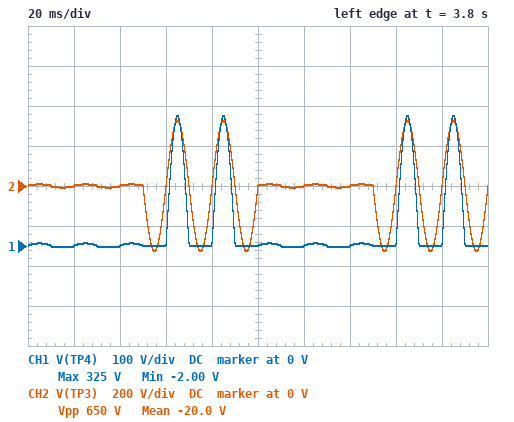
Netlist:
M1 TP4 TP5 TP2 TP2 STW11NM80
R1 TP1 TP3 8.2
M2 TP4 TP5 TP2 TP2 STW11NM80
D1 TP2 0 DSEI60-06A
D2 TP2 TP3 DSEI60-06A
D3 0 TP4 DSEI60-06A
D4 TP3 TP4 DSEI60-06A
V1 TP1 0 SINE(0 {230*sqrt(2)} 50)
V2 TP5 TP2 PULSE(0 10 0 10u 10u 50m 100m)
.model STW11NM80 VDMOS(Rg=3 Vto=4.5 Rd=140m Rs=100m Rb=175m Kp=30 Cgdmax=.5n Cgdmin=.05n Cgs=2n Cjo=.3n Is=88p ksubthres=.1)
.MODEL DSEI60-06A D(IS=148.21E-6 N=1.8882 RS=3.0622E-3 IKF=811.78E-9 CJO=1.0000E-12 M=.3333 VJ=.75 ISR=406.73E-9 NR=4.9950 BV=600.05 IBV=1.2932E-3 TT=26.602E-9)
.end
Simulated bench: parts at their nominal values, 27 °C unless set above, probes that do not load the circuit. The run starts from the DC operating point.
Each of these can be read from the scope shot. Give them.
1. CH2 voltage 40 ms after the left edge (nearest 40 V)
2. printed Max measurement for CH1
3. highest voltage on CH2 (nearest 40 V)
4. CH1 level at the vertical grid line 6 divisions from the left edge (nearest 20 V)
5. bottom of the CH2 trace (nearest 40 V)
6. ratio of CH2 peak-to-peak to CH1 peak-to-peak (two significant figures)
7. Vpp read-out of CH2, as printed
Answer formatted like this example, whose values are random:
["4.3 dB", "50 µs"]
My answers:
["0 V", "325 V", "320 V", "0 V", "-320 V", "2.0", "650 V"]
